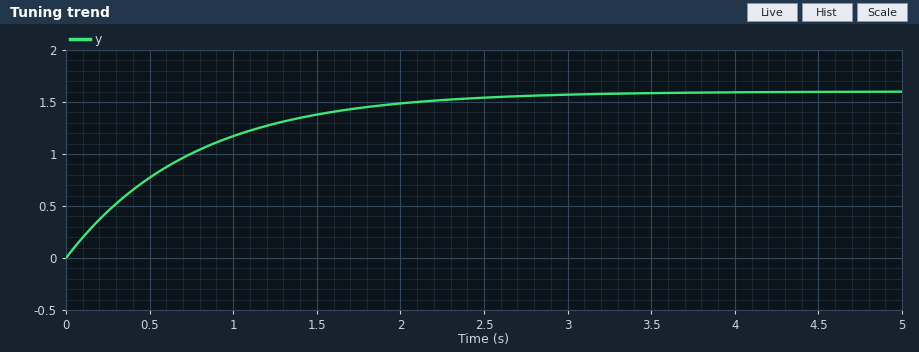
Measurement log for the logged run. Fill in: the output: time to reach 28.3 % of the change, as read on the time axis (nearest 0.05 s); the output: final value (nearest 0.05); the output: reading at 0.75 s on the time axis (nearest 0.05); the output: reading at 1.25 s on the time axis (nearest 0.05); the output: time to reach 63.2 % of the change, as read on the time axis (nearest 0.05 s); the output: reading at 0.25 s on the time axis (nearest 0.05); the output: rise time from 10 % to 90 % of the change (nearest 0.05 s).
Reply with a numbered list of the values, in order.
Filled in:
1. 0.25 s
2. 1.60
3. 1.00
4. 1.30
5. 0.75 s
6. 0.45
7. 1.65 s
